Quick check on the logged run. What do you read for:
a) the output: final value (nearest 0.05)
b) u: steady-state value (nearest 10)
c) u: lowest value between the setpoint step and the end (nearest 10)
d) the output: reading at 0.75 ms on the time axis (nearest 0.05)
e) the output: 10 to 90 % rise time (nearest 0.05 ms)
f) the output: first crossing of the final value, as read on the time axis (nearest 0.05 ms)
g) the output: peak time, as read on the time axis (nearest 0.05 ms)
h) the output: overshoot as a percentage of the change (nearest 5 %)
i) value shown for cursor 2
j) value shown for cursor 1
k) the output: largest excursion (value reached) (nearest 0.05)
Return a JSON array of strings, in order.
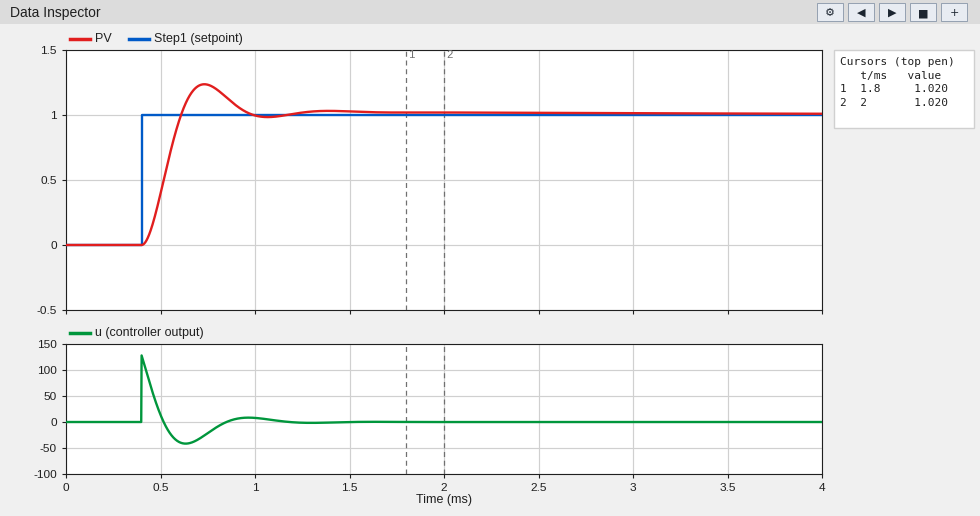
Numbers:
["1.00", "0", "-40", "1.25", "0.15 ms", "0.60 ms", "0.75 ms", "25 %", "1.020", "1.020", "1.25"]
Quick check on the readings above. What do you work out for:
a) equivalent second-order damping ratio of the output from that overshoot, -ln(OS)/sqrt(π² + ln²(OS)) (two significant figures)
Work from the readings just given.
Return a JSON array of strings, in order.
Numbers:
["0.40"]
